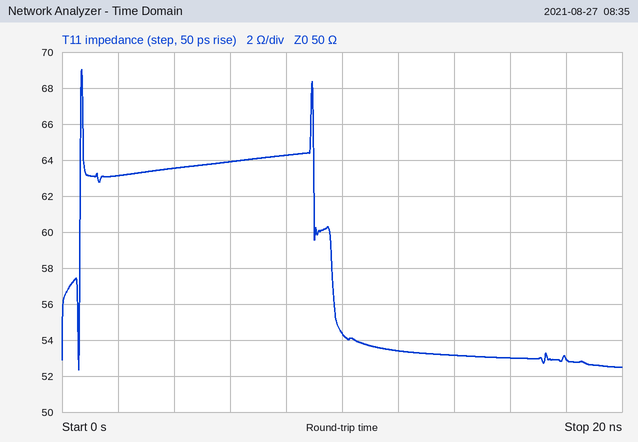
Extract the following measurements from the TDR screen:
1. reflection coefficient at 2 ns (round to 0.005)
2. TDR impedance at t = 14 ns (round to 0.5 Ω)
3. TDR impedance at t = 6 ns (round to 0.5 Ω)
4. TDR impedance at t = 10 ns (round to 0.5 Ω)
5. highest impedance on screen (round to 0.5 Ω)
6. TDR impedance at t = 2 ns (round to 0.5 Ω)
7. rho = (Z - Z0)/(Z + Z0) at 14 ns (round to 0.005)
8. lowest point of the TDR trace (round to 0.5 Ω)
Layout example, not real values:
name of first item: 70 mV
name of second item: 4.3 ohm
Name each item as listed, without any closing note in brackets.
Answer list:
reflection coefficient at 2 ns: +0.115
TDR impedance at t = 14 ns: 53.0 Ω
TDR impedance at t = 6 ns: 64.0 Ω
TDR impedance at t = 10 ns: 54.5 Ω
highest impedance on screen: 69.0 Ω
TDR impedance at t = 2 ns: 63.0 Ω
rho = (Z - Z0)/(Z + Z0) at 14 ns: +0.030
lowest point of the TDR trace: 52.5 Ω
